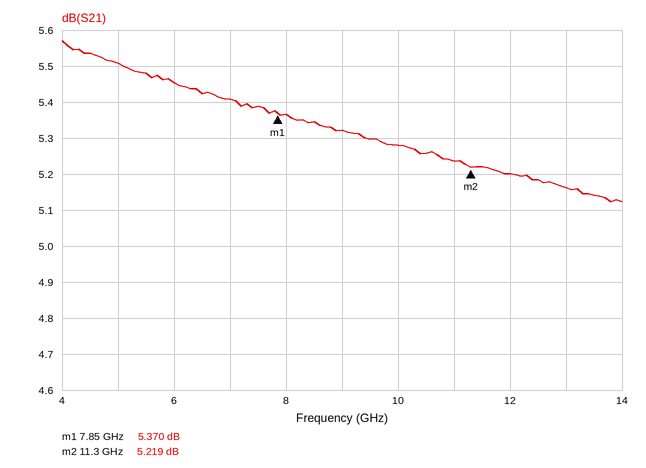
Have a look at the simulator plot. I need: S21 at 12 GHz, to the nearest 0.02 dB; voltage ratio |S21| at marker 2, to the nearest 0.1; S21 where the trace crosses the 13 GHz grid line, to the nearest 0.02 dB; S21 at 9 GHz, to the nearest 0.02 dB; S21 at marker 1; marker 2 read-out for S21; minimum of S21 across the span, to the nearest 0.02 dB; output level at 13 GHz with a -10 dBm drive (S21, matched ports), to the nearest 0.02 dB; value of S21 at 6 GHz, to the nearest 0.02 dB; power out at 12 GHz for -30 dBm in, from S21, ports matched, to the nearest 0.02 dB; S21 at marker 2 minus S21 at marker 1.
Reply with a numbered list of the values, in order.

1. 5.20 dB
2. 1.8
3. 5.16 dB
4. 5.32 dB
5. 5.370 dB
6. 5.219 dB
7. 5.12 dB
8. -4.84 dBm
9. 5.46 dB
10. -24.80 dBm
11. -0.151 dB
